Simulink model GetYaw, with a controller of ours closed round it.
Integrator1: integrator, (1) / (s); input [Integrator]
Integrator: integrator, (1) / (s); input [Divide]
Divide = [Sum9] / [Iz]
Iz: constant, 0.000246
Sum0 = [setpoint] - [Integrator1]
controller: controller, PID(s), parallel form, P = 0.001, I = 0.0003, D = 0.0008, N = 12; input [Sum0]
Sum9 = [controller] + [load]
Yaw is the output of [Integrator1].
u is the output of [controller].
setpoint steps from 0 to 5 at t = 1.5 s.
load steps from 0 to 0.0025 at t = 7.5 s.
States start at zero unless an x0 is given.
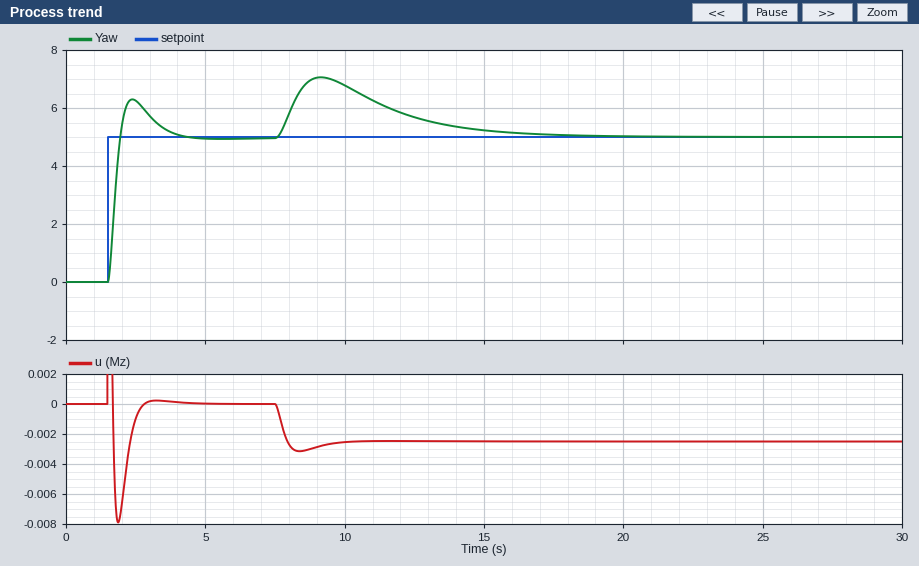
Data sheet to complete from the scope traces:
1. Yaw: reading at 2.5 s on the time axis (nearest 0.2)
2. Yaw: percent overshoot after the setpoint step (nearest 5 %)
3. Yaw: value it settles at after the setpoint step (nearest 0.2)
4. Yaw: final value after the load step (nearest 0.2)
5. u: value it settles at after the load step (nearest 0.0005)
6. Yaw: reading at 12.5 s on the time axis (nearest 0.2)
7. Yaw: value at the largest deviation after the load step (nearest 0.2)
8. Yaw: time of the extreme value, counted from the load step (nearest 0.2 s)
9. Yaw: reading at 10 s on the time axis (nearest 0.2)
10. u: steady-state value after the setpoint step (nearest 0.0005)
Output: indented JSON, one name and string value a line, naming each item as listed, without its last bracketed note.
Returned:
{
  "Yaw: reading at 2.5 s on the time axis": "6.2",
  "Yaw: percent overshoot after the setpoint step": "25 %",
  "Yaw: value it settles at after the setpoint step": "5.0",
  "Yaw: final value after the load step": "5.0",
  "u: value it settles at after the load step": "-0.0025",
  "Yaw: reading at 12.5 s on the time axis": "5.6",
  "Yaw: value at the largest deviation after the load step": "7.0",
  "Yaw: time of the extreme value, counted from the load step": "1.6 s",
  "Yaw: reading at 10 s on the time axis": "6.8",
  "u: steady-state value after the setpoint step": "0.0000"
}
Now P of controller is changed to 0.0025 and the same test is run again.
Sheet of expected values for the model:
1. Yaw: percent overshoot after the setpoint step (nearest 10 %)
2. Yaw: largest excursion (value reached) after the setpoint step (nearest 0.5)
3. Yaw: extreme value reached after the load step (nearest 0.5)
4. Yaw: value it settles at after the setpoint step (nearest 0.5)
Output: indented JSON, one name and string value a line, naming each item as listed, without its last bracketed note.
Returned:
{
  "Yaw: percent overshoot after the setpoint step": "40 %",
  "Yaw: largest excursion (value reached) after the setpoint step": "7.0",
  "Yaw: extreme value reached after the load step": "6.0",
  "Yaw: value it settles at after the setpoint step": "5.0"
}
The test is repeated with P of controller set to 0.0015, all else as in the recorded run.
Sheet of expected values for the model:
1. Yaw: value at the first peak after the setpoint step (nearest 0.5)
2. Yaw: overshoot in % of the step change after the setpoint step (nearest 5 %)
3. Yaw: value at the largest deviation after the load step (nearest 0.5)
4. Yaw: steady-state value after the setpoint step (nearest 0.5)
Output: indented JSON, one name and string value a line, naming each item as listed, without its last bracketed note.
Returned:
{
  "Yaw: value at the first peak after the setpoint step": "6.5",
  "Yaw: overshoot in % of the step change after the setpoint step": "30 %",
  "Yaw: value at the largest deviation after the load step": "6.5",
  "Yaw: steady-state value after the setpoint step": "5.0"
}
